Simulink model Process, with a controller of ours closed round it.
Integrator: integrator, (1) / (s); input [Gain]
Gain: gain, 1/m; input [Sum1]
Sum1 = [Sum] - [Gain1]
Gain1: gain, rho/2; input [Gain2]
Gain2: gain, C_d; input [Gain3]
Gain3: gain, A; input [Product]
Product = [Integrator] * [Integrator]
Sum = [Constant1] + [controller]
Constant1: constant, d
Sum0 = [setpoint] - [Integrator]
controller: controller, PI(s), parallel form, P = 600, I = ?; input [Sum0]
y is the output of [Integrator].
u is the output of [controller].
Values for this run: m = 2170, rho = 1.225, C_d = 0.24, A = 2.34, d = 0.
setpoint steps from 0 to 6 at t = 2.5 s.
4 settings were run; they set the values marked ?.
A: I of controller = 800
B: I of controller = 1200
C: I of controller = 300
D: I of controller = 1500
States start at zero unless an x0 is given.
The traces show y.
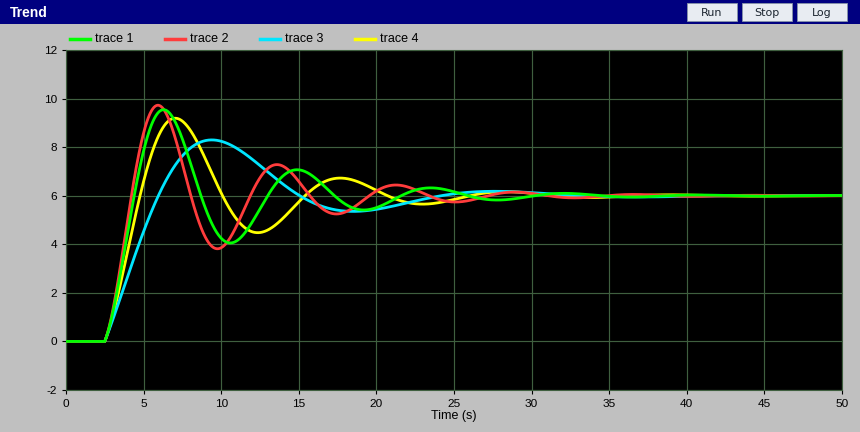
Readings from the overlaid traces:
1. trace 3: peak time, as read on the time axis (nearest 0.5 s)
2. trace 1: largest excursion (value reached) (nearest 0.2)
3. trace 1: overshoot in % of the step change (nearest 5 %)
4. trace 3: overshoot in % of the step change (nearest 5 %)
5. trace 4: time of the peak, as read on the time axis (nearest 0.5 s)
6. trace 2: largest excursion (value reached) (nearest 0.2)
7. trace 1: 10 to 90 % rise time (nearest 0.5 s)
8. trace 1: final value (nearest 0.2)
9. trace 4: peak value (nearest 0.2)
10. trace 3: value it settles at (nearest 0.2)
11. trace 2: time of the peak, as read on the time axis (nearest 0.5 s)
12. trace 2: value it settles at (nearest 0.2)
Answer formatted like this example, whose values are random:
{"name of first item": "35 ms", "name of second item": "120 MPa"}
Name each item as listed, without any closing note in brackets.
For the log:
{"trace 3: peak time, as read on the time axis": "9.5 s", "trace 1: largest excursion (value reached)": "9.6", "trace 1: overshoot in % of the step change": "60 %", "trace 3: overshoot in % of the step change": "40 %", "trace 4: time of the peak, as read on the time axis": "7.0 s", "trace 2: largest excursion (value reached)": "9.8", "trace 1: 10 to 90 % rise time": "1.5 s", "trace 1: final value": "6.0", "trace 4: peak value": "9.2", "trace 3: value it settles at": "6.0", "trace 2: time of the peak, as read on the time axis": "6.0 s", "trace 2: value it settles at": "6.0"}
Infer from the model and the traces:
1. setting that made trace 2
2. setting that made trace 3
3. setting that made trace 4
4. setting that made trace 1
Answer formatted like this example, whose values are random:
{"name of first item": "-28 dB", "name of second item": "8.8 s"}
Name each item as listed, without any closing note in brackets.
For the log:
{"setting that made trace 2": "D", "setting that made trace 3": "C", "setting that made trace 4": "A", "setting that made trace 1": "B"}
